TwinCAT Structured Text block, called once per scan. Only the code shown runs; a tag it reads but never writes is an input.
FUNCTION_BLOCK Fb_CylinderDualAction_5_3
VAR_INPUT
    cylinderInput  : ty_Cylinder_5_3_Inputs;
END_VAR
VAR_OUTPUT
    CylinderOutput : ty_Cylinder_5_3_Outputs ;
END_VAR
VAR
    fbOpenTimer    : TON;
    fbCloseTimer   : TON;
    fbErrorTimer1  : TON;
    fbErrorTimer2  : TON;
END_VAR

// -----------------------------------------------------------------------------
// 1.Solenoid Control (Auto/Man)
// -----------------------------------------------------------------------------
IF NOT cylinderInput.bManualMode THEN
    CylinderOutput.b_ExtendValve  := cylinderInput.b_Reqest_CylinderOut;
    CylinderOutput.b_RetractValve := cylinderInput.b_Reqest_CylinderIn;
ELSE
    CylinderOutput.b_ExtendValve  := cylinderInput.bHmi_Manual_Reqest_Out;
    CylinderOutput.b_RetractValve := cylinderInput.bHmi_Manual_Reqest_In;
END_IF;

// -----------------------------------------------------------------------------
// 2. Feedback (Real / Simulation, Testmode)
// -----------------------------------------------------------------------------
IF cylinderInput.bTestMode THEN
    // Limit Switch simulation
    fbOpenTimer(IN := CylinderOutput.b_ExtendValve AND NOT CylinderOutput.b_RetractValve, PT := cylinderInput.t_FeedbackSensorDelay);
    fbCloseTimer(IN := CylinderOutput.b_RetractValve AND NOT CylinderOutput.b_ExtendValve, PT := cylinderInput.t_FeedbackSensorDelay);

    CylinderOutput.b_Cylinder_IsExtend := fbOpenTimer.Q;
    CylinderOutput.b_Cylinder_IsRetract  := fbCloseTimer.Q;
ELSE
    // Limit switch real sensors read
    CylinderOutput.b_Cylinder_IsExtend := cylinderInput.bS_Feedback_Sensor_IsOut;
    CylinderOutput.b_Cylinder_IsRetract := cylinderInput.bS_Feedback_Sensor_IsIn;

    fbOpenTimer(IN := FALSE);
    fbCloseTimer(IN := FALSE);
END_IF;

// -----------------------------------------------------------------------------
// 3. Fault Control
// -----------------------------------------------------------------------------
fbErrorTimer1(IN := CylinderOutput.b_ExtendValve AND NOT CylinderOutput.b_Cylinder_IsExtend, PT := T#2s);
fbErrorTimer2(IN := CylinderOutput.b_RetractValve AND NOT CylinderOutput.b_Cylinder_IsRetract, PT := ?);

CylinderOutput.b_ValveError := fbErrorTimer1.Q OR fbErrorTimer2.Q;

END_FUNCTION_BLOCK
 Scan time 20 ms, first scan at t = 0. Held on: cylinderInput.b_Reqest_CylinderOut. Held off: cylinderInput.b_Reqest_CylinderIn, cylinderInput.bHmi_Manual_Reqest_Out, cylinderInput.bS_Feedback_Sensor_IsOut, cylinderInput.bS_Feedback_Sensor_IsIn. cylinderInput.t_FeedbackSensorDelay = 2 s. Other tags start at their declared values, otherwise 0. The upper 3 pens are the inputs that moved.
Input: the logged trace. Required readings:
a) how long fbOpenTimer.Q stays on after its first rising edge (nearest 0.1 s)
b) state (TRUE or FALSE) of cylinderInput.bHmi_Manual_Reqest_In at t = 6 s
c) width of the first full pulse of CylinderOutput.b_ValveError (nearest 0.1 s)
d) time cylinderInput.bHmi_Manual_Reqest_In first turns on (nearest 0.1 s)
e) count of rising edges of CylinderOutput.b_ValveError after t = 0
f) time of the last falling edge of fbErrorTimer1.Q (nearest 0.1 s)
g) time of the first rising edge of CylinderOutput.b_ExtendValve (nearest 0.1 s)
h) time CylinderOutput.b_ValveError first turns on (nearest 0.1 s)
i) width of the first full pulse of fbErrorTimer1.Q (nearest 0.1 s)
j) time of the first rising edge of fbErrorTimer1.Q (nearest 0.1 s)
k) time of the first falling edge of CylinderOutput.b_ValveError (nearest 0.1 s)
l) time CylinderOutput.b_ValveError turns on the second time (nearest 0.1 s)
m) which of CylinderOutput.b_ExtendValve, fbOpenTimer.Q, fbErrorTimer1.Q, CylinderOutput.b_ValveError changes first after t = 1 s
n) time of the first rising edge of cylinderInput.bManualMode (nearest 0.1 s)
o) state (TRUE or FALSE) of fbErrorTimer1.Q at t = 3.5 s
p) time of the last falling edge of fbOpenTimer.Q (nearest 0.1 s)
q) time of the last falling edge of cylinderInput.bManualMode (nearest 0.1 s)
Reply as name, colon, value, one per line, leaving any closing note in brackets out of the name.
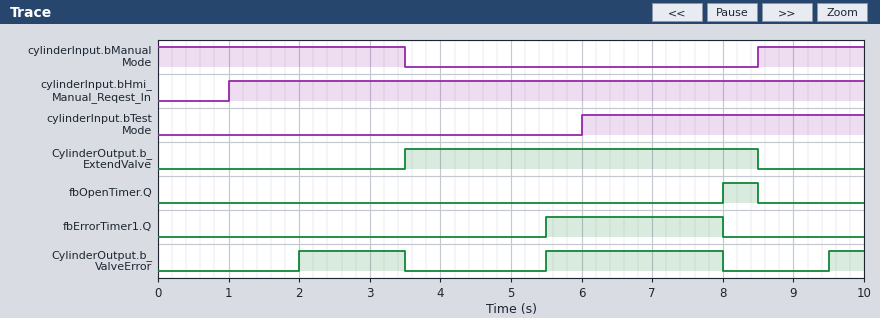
how long fbOpenTimer.Q stays on after its first rising edge: 0.5 s
state (TRUE or FALSE) of cylinderInput.bHmi_Manual_Reqest_In at t = 6 s: TRUE
width of the first full pulse of CylinderOutput.b_ValveError: 1.5 s
time cylinderInput.bHmi_Manual_Reqest_In first turns on: 1.0 s
count of rising edges of CylinderOutput.b_ValveError after t = 0: 3
time of the last falling edge of fbErrorTimer1.Q: 8.0 s
time of the first rising edge of CylinderOutput.b_ExtendValve: 3.5 s
time CylinderOutput.b_ValveError first turns on: 2.0 s
width of the first full pulse of fbErrorTimer1.Q: 2.5 s
time of the first rising edge of fbErrorTimer1.Q: 5.5 s
time of the first falling edge of CylinderOutput.b_ValveError: 3.5 s
time CylinderOutput.b_ValveError turns on the second time: 5.5 s
which of CylinderOutput.b_ExtendValve, fbOpenTimer.Q, fbErrorTimer1.Q, CylinderOutput.b_ValveError changes first after t = 1 s: CylinderOutput.b_ValveError
time of the first rising edge of cylinderInput.bManualMode: 8.5 s
state (TRUE or FALSE) of fbErrorTimer1.Q at t = 3.5 s: FALSE
time of the last falling edge of fbOpenTimer.Q: 8.5 s
time of the last falling edge of cylinderInput.bManualMode: 3.5 s
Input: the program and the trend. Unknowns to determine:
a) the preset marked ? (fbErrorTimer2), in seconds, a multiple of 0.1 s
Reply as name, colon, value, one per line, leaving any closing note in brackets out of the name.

the preset marked ? (fbErrorTimer2), in seconds, a multiple of 0.1 s: 1.0 s
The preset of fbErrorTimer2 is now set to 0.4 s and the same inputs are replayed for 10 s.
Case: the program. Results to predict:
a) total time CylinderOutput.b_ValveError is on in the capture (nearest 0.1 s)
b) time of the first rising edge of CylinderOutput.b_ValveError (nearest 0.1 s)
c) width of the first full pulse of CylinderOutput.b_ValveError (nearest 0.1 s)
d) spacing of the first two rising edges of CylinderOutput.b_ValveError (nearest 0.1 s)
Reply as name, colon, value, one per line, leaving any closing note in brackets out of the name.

total time CylinderOutput.b_ValveError is on in the capture: 5.7 s
time of the first rising edge of CylinderOutput.b_ValveError: 1.4 s
width of the first full pulse of CylinderOutput.b_ValveError: 2.1 s
spacing of the first two rising edges of CylinderOutput.b_ValveError: 4.1 s
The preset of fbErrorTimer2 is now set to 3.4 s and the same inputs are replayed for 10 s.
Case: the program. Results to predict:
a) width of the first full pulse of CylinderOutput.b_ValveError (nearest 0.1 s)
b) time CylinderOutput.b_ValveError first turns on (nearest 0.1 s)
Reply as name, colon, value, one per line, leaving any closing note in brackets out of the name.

width of the first full pulse of CylinderOutput.b_ValveError: 2.5 s
time CylinderOutput.b_ValveError first turns on: 5.5 s
